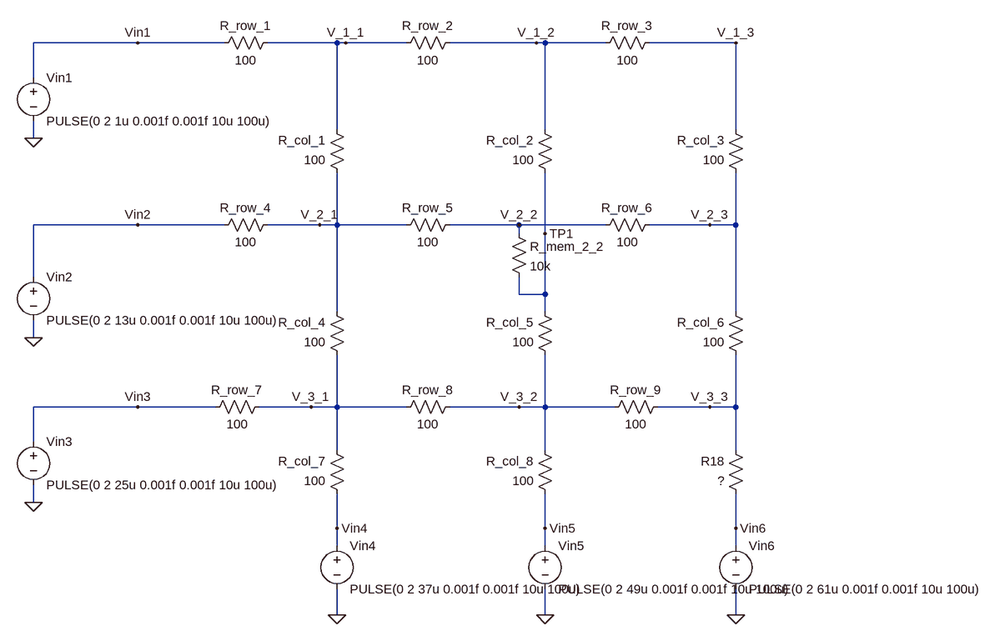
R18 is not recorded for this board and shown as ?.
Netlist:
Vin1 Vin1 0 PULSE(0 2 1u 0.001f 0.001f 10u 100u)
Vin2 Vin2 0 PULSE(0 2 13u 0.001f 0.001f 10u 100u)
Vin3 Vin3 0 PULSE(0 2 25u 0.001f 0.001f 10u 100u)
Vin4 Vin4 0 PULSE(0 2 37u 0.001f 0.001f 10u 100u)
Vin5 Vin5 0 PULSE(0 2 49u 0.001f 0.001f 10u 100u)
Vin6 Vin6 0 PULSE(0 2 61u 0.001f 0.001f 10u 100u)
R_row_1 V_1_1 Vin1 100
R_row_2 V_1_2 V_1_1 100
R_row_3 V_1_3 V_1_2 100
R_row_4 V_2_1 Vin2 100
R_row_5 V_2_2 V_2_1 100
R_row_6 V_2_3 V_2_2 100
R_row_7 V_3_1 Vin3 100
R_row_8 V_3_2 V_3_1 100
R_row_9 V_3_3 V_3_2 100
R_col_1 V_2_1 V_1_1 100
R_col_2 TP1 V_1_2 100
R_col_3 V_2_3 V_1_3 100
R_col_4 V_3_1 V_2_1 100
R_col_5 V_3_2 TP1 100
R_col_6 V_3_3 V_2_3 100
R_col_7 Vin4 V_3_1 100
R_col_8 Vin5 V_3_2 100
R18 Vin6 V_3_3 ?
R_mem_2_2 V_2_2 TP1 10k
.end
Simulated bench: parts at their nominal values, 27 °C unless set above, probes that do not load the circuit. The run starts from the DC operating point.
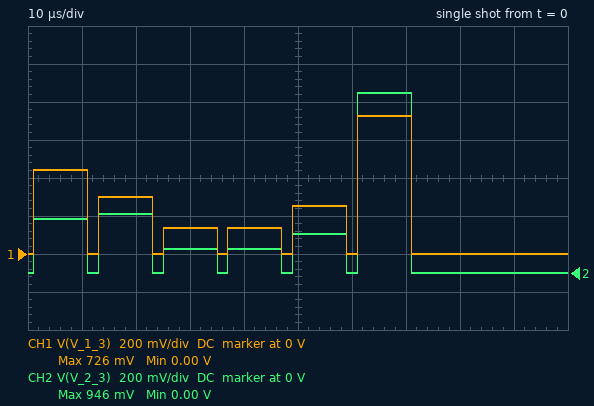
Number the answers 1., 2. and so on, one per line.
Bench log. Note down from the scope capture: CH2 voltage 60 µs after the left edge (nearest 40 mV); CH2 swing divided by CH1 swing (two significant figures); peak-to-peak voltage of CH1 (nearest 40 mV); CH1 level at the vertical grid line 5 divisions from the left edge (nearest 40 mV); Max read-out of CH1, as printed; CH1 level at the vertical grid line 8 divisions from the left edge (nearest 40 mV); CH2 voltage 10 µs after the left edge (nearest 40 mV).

1. 0 V
2. 1.3
3. 720 mV
4. 240 mV
5. 726 mV
6. 0 V
7. 280 mV
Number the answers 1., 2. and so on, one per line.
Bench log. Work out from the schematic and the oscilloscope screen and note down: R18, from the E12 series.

1. 33 Ω
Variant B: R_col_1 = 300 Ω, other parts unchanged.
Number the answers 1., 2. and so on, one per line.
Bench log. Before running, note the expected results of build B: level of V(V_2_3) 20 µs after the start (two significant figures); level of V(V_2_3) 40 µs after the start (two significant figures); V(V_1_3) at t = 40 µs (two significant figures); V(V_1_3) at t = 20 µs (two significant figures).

1. 320 mV
2. 130 mV
3. 130 mV
4. 270 mV
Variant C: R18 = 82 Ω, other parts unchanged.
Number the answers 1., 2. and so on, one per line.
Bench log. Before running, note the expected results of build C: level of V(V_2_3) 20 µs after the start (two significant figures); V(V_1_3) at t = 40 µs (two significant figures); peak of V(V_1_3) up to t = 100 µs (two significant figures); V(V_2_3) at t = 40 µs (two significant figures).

1. 360 mV
2. 170 mV
3. 530 mV
4. 160 mV
